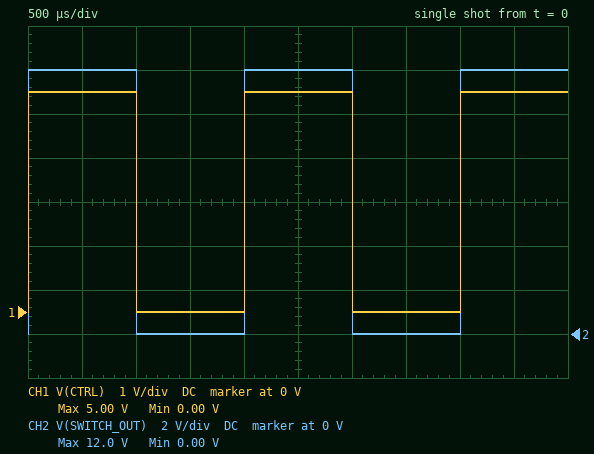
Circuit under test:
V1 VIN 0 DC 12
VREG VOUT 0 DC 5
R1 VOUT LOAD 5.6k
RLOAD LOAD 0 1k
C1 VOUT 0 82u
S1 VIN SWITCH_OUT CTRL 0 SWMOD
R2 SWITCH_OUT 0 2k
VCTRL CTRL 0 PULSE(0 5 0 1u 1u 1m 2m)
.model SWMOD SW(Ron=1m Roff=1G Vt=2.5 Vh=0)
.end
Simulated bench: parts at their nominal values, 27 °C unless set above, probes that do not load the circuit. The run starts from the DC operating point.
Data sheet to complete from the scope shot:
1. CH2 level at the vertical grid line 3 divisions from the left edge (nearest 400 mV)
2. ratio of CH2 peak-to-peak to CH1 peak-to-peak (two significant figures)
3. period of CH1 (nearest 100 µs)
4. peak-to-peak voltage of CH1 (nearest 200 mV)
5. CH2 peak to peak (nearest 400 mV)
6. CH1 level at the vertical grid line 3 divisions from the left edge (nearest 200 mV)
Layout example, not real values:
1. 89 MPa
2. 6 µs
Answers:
1. 0 V
2. 2.4
3. 2.0 ms
4. 5.0 V
5. 12.0 V
6. 0 V
